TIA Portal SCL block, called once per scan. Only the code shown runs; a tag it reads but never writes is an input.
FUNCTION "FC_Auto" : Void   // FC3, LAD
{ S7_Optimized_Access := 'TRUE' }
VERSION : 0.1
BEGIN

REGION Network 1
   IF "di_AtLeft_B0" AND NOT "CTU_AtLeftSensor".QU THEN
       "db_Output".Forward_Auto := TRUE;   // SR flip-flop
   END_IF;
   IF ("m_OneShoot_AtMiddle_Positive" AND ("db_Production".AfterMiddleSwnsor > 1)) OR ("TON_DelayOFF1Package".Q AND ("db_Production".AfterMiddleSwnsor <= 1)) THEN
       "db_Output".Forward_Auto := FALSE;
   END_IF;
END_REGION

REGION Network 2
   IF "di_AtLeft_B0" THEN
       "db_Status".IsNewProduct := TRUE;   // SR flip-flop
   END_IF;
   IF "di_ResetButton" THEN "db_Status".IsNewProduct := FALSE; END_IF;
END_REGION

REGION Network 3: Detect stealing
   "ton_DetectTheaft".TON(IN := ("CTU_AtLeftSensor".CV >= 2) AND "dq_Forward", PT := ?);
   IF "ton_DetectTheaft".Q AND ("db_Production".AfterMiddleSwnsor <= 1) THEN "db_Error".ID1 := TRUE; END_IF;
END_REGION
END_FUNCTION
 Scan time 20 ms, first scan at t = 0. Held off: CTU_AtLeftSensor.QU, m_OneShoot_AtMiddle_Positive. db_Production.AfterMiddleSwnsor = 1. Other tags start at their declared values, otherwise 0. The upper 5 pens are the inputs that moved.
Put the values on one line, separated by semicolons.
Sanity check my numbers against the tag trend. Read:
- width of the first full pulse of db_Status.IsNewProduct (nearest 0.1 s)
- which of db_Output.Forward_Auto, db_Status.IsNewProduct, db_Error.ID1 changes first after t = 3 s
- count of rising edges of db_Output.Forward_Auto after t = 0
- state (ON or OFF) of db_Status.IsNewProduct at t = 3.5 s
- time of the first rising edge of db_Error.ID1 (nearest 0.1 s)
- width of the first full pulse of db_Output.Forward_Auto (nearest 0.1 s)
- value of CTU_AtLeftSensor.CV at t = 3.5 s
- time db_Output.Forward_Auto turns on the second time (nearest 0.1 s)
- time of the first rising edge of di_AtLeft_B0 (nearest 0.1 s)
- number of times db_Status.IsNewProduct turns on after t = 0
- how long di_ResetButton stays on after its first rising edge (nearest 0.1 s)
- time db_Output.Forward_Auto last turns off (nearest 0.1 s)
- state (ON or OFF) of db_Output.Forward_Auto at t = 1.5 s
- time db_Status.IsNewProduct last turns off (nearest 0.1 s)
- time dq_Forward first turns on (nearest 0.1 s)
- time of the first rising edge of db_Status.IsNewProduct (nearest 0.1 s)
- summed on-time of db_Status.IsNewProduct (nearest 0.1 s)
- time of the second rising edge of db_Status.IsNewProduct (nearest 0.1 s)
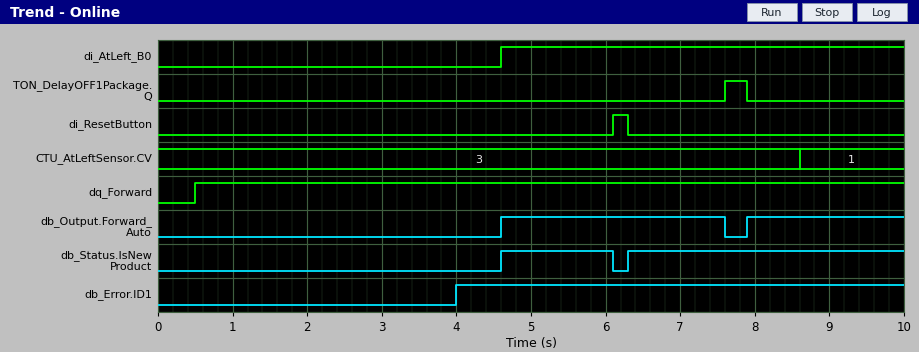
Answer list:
1.5 s; db_Error.ID1; 2; OFF; 4.0 s; 3.0 s; 3; 7.9 s; 4.6 s; 2; 0.2 s; 7.6 s; OFF; 6.1 s; 0.5 s; 4.6 s; 5.2 s; 6.3 s
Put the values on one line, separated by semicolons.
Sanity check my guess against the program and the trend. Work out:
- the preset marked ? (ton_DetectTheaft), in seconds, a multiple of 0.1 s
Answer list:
3.5 s
